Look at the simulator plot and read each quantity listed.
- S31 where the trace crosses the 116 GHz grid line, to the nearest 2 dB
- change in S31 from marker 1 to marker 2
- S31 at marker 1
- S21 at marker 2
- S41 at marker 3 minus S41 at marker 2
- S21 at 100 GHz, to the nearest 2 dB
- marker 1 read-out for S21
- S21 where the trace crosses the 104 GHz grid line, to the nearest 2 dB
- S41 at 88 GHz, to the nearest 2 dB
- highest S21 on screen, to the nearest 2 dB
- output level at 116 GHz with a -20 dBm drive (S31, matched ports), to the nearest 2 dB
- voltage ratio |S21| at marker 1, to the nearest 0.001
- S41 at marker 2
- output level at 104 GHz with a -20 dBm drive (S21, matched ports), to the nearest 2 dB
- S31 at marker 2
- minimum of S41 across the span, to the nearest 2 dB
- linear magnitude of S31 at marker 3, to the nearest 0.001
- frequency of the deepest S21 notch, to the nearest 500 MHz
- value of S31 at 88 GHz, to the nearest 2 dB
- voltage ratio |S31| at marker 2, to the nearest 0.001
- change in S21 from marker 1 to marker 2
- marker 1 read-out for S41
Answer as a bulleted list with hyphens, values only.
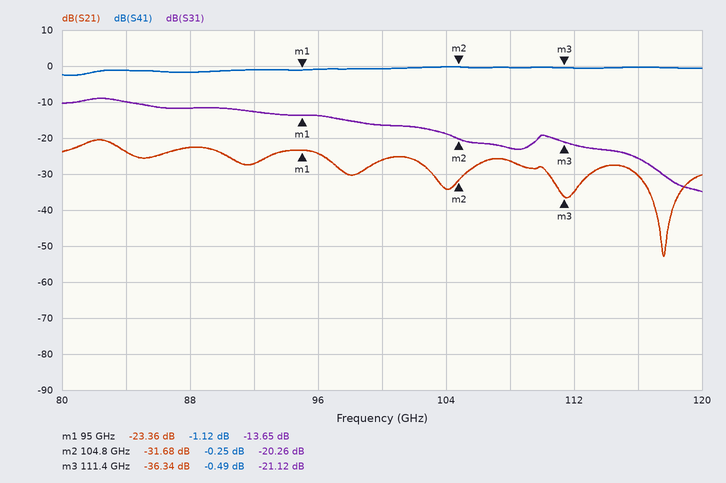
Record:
- -26 dB
- -6.61 dB
- -13.65 dB
- -31.68 dB
- -0.24 dB
- -26 dB
- -23.36 dB
- -34 dB
- -2 dB
- -20 dB
- -46 dBm
- 0.068
- -0.25 dB
- -54 dBm
- -20.26 dB
- -2 dB
- 0.088
- 117.5 GHz
- -12 dB
- 0.097
- -8.32 dB
- -1.12 dB
